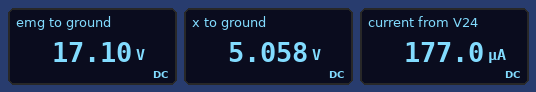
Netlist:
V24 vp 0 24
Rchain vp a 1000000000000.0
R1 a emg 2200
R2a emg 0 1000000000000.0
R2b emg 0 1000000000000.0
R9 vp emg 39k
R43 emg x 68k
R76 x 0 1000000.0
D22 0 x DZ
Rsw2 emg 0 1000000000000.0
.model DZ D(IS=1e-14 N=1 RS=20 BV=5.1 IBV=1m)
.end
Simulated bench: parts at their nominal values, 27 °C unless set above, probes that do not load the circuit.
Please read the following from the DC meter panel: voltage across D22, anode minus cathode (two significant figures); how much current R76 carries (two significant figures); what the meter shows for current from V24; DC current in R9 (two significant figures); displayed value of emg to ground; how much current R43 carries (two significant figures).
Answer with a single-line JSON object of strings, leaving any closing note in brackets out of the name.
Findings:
{"voltage across D22, anode minus cathode": "-5.1 V", "how much current R76 carries": "5.1 µA", "what the meter shows for current from V24": "177.0 µA", "DC current in R9": "180 µA", "displayed value of emg to ground": "17.10 V", "how much current R43 carries": "180 µA"}
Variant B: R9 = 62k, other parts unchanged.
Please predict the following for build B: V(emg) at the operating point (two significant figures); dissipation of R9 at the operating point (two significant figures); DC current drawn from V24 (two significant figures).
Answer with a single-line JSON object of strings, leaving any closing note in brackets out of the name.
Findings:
{"V(emg) at the operating point": "15 V", "dissipation of R9 at the operating point": "1.3 mW", "DC current drawn from V24": "150 µA"}
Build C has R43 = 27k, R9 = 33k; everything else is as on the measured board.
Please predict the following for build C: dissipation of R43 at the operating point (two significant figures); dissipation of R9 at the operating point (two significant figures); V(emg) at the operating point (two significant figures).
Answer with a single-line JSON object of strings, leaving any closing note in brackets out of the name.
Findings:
{"dissipation of R43 at the operating point": "2.7 mW", "dissipation of R9 at the operating point": "3.3 mW", "V(emg) at the operating point": "14 V"}
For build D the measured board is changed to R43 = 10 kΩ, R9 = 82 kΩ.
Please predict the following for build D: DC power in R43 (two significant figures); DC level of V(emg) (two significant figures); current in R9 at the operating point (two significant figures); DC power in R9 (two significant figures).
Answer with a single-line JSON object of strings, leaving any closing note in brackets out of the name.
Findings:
{"DC power in R43": "420 µW", "DC level of V(emg)": "7.1 V", "current in R9 at the operating point": "210 µA", "DC power in R9": "3.5 mW"}
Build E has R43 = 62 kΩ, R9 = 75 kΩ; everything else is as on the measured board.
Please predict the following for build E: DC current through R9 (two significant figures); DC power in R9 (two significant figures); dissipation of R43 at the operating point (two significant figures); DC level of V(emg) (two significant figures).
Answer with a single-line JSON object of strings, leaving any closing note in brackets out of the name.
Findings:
{"DC current through R9": "140 µA", "DC power in R9": "1.4 mW", "dissipation of R43 at the operating point": "1.2 mW", "DC level of V(emg)": "14 V"}
